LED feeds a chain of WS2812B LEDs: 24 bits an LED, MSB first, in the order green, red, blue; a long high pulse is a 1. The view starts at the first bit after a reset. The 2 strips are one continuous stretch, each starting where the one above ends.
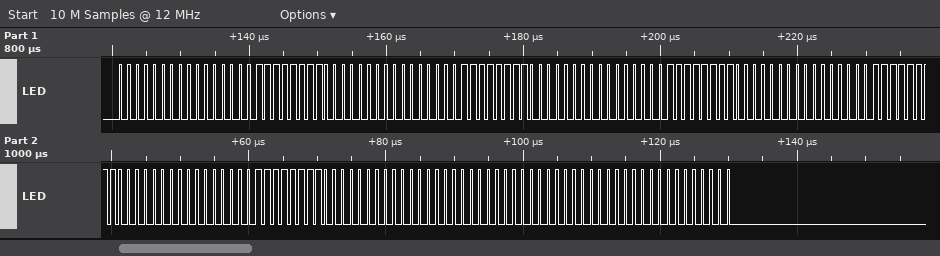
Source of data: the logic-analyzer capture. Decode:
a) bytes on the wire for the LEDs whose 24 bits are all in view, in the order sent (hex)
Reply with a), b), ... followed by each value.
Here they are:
a) 00 00 FF 00 00 FF 00 00 FF 00 00 FF 00 00 FF 00 00 00 00 00 00
